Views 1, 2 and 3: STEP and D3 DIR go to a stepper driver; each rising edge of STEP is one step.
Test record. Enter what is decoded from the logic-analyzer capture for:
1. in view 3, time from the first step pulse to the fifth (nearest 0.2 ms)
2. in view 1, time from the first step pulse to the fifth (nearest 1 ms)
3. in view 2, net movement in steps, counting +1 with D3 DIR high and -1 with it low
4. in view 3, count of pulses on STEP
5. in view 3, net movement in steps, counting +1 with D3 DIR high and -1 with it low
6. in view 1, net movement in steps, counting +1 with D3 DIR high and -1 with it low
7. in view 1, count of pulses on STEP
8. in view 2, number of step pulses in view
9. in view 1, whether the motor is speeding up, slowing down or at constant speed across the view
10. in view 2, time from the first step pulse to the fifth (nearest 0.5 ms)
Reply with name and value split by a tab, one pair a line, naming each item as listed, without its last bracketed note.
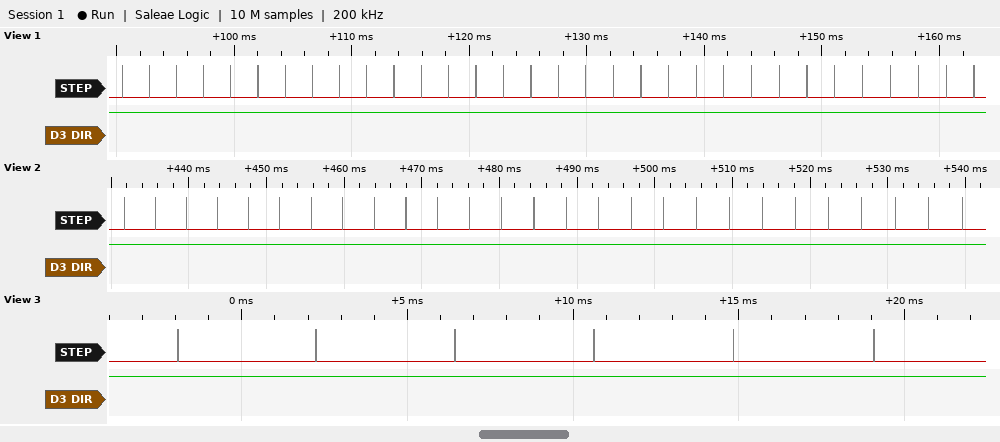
in view 3, time from the first step pulse to the fifth	16.8 ms
in view 1, time from the first step pulse to the fifth	9 ms
in view 2, net movement in steps, counting +1 with D3 DIR high and -1 with it low	+27
in view 3, count of pulses on STEP	6
in view 3, net movement in steps, counting +1 with D3 DIR high and -1 with it low	+6
in view 1, net movement in steps, counting +1 with D3 DIR high and -1 with it low	+32
in view 1, count of pulses on STEP	32
in view 2, number of step pulses in view	27
in view 1, whether the motor is speeding up, slowing down or at constant speed across the view	constant speed
in view 2, time from the first step pulse to the fifth	16.0 ms
